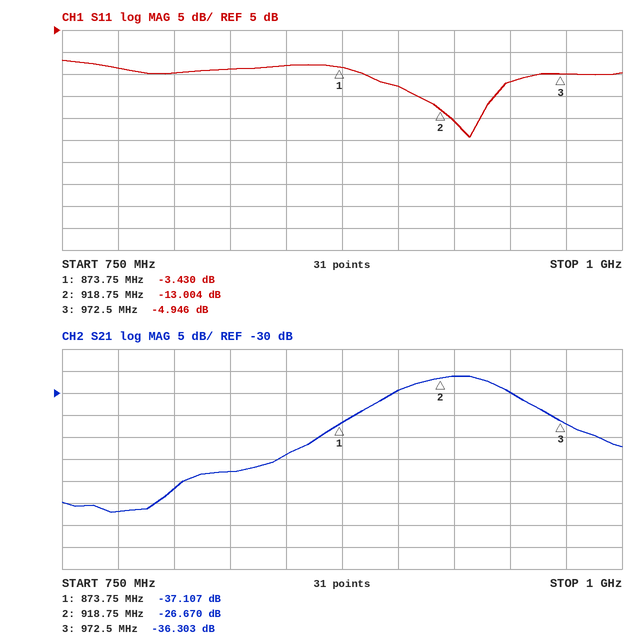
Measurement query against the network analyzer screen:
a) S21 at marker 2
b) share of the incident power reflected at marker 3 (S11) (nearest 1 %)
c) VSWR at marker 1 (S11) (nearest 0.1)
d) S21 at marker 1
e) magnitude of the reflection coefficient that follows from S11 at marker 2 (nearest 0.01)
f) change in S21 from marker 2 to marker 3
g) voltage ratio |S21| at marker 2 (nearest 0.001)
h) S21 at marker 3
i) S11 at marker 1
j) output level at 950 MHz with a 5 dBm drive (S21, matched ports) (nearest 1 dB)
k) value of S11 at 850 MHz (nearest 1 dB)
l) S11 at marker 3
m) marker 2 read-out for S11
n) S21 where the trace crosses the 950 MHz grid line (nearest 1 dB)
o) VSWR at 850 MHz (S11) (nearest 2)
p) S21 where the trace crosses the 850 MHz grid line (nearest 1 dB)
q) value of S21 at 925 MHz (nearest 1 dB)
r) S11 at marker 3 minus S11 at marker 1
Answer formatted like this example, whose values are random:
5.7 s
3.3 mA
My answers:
-26.670 dB
32 %
5.1
-37.107 dB
0.22
-9.633 dB
0.046
-36.303 dB
-3.430 dB
-25 dBm
-3 dB
-4.946 dB
-13.004 dB
-30 dB
6
-44 dB
-26 dB
-1.516 dB
